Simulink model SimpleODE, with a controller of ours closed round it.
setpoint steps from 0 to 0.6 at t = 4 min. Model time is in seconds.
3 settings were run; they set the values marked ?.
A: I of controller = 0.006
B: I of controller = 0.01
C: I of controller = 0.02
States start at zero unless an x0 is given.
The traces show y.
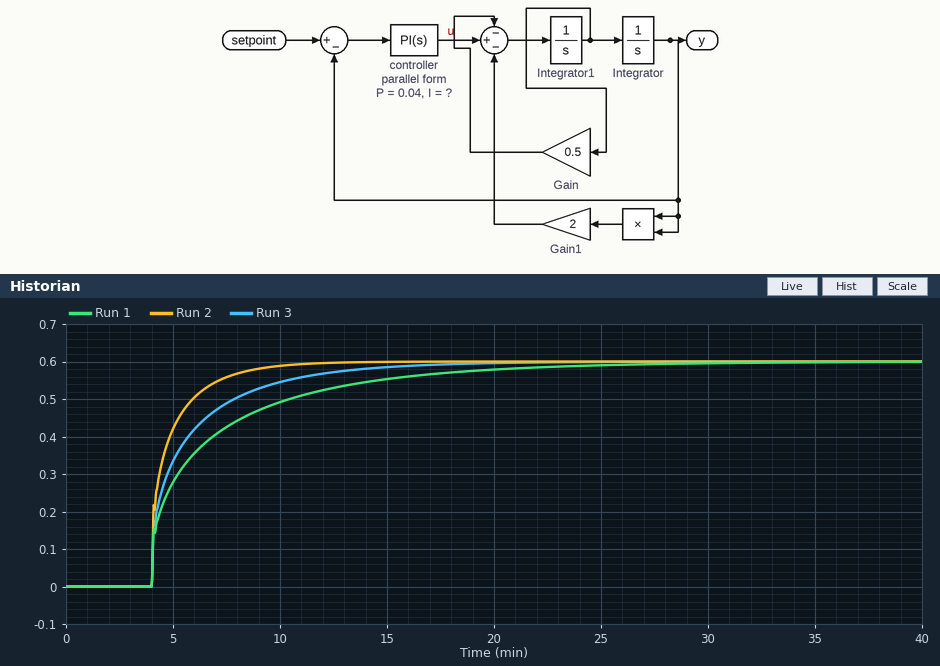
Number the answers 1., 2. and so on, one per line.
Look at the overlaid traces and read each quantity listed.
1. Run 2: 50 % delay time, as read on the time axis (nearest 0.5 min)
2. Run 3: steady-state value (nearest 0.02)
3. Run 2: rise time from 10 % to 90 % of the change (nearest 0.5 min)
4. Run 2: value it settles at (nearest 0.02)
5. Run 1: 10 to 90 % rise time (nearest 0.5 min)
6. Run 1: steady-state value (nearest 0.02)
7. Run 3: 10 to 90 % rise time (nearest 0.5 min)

1. 4.5 min
2. 0.60
3. 3.0 min
4. 0.60
5. 9.5 min
6. 0.60
7. 5.5 min
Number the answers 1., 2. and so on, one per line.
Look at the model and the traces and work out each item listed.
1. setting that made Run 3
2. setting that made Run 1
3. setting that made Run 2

1. B
2. A
3. C
